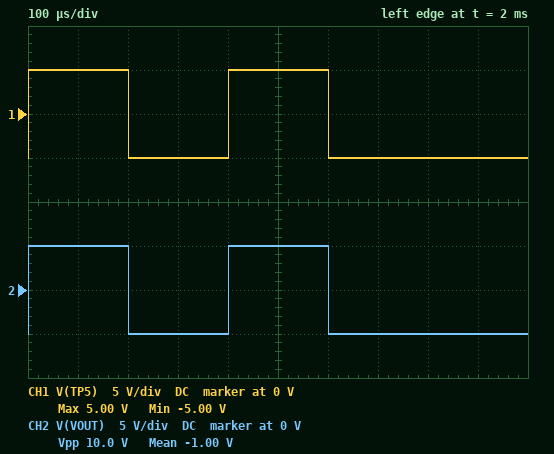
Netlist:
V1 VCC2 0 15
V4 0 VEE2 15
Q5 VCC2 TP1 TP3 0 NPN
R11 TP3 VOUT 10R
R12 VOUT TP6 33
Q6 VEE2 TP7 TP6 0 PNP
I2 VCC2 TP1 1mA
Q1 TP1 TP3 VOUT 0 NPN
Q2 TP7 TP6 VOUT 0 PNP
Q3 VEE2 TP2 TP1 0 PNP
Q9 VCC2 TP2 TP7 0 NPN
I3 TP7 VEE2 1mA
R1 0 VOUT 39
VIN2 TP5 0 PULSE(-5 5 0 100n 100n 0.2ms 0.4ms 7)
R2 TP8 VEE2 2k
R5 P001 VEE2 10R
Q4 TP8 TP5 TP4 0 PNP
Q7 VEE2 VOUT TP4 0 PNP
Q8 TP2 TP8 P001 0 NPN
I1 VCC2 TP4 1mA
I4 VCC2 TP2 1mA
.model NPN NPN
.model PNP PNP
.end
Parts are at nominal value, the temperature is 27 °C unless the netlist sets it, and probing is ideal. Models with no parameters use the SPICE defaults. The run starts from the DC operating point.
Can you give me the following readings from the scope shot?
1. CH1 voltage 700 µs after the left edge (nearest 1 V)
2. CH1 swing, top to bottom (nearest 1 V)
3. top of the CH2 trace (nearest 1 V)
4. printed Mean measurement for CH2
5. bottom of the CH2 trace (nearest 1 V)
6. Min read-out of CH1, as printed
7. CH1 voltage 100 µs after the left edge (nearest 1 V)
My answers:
-5 V
10 V
5 V
-1.00 V
-5 V
-5.00 V
5 V
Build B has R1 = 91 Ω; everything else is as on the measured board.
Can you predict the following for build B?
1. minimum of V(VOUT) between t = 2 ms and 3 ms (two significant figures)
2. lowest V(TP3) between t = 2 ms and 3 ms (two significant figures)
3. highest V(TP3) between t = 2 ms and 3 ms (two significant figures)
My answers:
-5.0 V
-5.2 V
5.5 V
